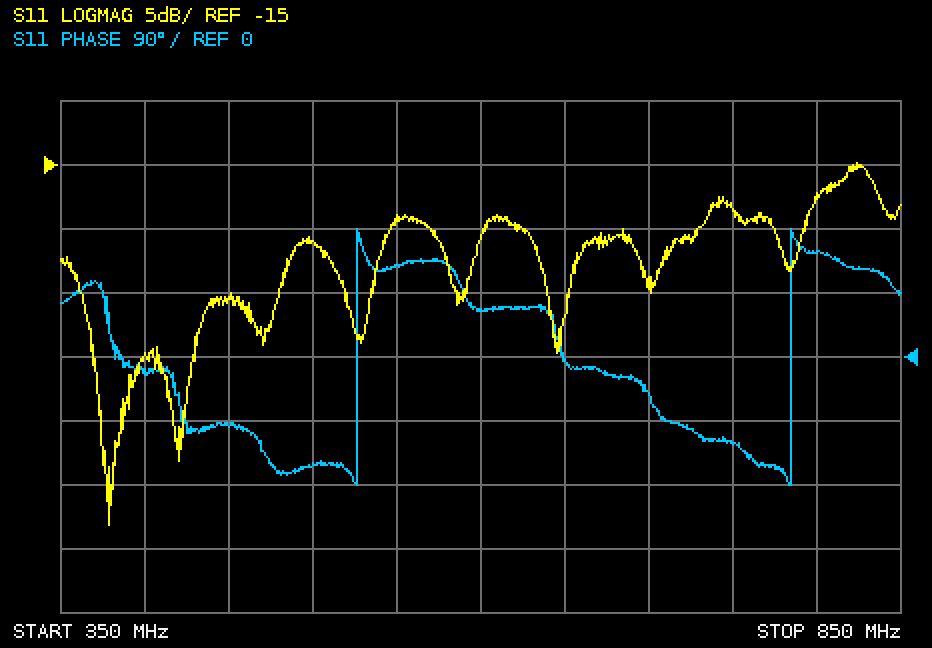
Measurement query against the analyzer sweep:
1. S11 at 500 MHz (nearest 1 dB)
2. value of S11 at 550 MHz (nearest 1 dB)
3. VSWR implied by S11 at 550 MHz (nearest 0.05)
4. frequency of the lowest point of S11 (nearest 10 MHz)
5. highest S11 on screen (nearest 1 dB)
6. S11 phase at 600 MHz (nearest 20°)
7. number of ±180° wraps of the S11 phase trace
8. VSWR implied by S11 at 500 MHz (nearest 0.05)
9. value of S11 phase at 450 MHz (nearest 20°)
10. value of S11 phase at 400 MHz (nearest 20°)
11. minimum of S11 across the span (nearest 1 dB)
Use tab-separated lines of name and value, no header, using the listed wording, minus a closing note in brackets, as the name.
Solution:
S11 at 500 MHz	-21 dB
value of S11 at 550 MHz	-19 dB
VSWR implied by S11 at 550 MHz	1.25
frequency of the lowest point of S11	380 MHz
highest S11 on screen	-15 dB
S11 phase at 600 MHz	60°
number of ±180° wraps of the S11 phase trace	2
VSWR implied by S11 at 500 MHz	1.20
value of S11 phase at 450 MHz	-100°
value of S11 phase at 400 MHz	-20°
minimum of S11 across the span	-43 dB
